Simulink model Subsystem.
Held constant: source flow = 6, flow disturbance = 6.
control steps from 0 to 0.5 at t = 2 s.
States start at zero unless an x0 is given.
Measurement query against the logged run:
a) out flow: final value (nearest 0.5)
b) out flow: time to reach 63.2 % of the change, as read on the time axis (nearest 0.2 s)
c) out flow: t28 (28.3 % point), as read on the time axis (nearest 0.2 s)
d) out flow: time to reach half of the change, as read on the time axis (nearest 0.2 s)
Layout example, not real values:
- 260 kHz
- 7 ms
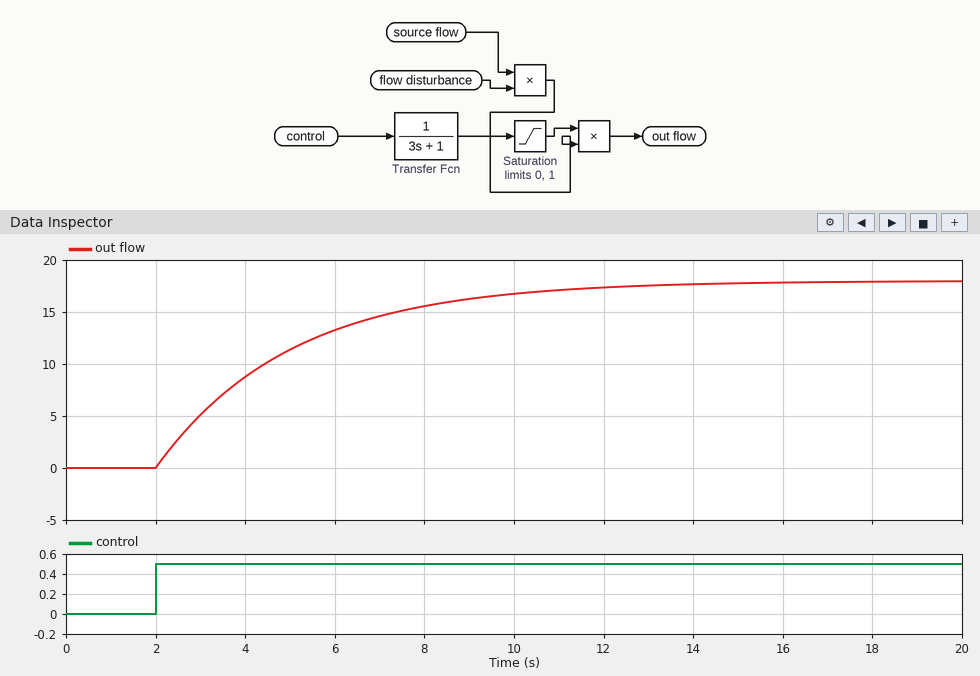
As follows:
- 18.0
- 5.0 s
- 3.0 s
- 4.0 s
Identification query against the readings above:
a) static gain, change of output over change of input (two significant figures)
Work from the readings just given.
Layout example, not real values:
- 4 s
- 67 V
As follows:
- 36
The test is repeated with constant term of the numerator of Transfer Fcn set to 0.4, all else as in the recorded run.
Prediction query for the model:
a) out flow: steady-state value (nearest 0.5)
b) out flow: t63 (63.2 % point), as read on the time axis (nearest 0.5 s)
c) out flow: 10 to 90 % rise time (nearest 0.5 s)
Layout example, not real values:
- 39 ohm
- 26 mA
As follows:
- 7.0
- 5.0 s
- 6.5 s
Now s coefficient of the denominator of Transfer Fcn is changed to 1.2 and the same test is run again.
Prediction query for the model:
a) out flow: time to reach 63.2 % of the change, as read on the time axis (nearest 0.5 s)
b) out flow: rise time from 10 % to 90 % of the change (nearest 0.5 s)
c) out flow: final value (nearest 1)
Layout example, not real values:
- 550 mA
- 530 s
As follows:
- 3.0 s
- 2.5 s
- 18
